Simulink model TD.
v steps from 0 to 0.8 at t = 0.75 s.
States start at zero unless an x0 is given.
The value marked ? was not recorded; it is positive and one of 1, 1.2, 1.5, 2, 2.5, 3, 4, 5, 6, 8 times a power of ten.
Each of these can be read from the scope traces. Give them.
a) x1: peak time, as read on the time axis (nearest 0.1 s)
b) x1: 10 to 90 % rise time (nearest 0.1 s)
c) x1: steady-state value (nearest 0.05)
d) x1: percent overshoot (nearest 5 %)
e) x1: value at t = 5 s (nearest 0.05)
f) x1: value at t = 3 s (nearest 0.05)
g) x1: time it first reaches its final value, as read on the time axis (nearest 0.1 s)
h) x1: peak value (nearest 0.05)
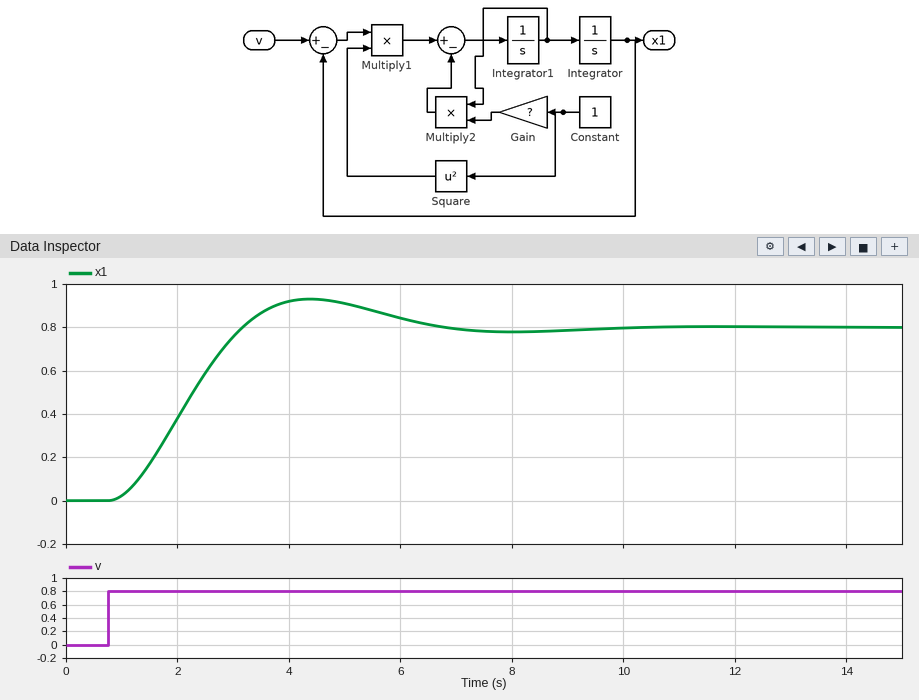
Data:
4.4 s
1.6 s
0.80
15 %
0.90
0.75
3.2 s
0.95
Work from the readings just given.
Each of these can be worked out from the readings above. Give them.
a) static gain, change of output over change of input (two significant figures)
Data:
1.0
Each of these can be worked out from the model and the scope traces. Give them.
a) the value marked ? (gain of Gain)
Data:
1
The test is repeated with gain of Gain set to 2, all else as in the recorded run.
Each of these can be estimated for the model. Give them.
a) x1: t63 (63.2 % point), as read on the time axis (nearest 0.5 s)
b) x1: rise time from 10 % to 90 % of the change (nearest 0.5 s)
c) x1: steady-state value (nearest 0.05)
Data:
3.0 s
3.5 s
0.80
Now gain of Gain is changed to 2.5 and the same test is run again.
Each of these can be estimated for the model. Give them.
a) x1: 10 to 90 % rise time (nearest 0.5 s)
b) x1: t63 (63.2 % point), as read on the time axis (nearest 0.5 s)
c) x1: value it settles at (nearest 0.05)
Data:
4.5 s
3.5 s
0.80
